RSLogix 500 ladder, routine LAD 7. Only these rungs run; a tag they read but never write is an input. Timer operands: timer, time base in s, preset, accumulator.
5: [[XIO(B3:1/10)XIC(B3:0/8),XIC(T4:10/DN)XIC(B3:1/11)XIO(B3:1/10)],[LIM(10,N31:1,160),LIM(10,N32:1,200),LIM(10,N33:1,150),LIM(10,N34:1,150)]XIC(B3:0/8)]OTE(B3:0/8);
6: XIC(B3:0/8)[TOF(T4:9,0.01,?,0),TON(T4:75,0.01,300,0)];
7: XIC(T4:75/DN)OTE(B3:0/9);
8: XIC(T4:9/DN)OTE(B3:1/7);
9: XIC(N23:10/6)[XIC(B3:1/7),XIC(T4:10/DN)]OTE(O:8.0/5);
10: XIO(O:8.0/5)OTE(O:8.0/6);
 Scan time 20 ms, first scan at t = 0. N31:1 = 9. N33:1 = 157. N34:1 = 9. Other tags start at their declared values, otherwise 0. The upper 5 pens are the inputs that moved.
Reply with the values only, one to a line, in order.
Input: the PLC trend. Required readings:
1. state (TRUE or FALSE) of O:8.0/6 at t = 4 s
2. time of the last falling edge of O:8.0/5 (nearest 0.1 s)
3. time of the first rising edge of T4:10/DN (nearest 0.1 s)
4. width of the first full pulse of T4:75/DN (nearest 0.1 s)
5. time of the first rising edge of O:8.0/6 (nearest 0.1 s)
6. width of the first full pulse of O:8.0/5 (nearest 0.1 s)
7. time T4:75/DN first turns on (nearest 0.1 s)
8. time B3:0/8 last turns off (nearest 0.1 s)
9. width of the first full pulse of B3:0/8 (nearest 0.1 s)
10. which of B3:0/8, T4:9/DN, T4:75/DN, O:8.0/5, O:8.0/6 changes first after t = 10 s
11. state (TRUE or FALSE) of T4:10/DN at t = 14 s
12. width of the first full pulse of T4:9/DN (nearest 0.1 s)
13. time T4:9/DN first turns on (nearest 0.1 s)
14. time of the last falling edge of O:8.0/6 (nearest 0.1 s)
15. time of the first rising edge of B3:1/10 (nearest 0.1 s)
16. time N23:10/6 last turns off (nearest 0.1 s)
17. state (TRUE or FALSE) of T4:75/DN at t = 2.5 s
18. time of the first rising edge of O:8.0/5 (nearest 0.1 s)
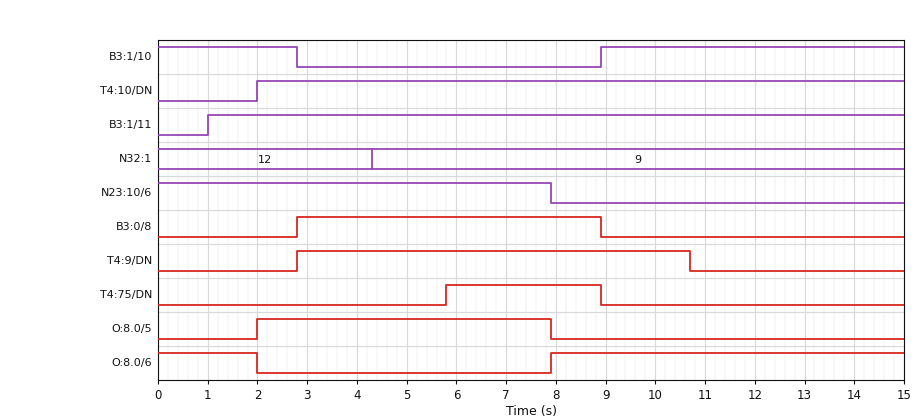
FALSE
7.9 s
2.0 s
3.1 s
7.9 s
5.9 s
5.8 s
8.9 s
6.1 s
T4:9/DN
TRUE
7.9 s
2.8 s
2.0 s
8.9 s
7.9 s
FALSE
2.0 s
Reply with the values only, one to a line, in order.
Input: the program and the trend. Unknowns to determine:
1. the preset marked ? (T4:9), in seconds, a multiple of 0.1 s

1.8 s
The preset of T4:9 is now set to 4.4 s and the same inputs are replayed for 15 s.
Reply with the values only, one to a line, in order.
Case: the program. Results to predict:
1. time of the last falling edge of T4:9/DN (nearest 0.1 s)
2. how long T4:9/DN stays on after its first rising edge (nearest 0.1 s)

13.3 s
10.5 s
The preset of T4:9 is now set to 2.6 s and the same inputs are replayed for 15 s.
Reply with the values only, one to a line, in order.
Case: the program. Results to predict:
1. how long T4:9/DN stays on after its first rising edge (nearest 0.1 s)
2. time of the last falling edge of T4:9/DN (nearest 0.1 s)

8.7 s
11.5 s
